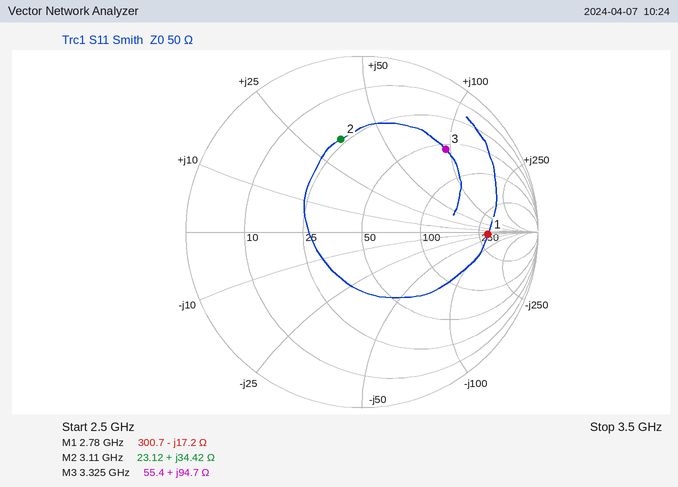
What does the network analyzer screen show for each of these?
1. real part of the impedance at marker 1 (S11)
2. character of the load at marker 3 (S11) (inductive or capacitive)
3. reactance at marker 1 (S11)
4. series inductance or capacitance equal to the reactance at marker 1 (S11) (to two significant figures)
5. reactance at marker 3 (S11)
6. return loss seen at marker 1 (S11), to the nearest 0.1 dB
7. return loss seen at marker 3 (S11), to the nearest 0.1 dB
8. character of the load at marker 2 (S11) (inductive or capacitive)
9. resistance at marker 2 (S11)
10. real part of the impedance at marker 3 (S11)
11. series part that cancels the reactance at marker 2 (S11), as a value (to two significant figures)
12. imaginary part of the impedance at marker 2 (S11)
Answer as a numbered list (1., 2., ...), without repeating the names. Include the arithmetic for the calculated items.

1. 300.7 Ω
2. inductive
3. -17.2 Ω
4. C = 1/(2π × 2.78 GHz × 17.2 Ω) ≈ 3.3 pF
5. +94.7 Ω
6. 2.9 dB
7. 3.5 dB
8. inductive
9. 23.12 Ω
10. 55.4 Ω
11. C = 1/(2π × 3.11 GHz × 34.42 Ω) ≈ 1.5 pF
12. +34.42 Ω
